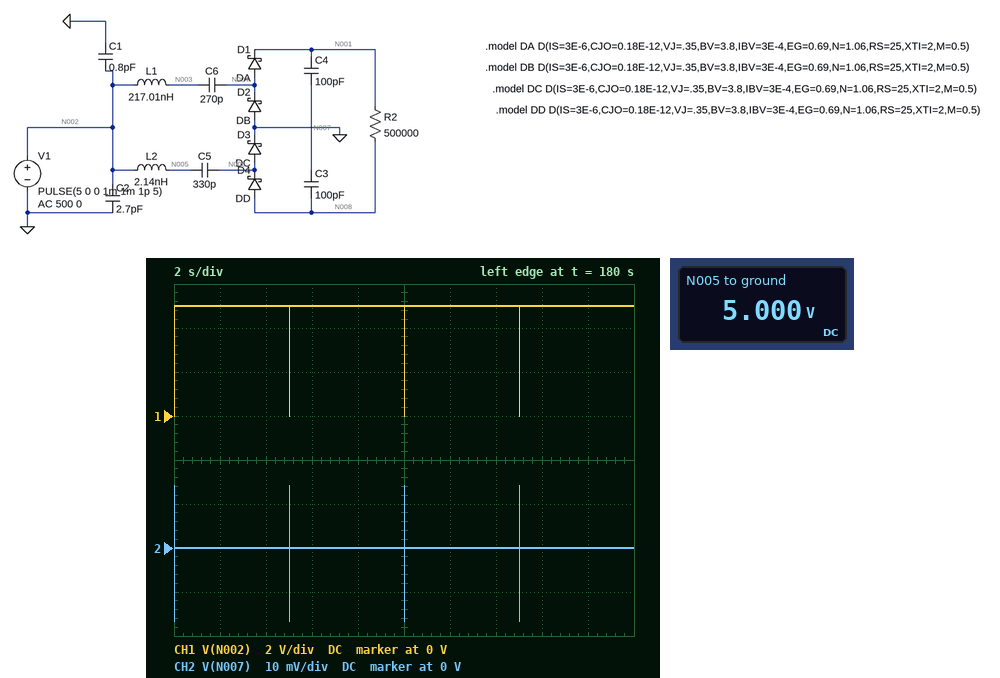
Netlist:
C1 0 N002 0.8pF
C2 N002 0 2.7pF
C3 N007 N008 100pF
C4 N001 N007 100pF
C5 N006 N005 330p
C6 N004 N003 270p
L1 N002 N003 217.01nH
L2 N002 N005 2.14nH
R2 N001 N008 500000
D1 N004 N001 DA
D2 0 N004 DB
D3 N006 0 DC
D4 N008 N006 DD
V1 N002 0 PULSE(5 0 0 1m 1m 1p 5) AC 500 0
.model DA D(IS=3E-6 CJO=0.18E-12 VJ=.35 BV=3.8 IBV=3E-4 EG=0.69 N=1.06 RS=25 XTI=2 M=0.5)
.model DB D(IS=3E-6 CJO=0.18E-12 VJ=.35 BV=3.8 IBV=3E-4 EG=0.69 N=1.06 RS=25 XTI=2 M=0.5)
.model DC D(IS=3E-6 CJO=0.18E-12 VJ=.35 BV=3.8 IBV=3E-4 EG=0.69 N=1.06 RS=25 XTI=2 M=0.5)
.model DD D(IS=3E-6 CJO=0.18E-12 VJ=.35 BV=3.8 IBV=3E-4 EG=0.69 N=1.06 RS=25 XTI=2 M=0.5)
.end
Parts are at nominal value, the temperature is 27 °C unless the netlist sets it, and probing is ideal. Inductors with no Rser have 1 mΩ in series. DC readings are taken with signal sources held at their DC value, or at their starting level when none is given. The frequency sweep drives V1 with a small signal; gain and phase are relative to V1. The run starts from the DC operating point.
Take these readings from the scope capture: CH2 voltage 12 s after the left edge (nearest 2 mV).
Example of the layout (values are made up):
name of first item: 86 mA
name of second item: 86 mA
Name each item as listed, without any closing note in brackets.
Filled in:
CH2 voltage 12 s after the left edge: 0 V
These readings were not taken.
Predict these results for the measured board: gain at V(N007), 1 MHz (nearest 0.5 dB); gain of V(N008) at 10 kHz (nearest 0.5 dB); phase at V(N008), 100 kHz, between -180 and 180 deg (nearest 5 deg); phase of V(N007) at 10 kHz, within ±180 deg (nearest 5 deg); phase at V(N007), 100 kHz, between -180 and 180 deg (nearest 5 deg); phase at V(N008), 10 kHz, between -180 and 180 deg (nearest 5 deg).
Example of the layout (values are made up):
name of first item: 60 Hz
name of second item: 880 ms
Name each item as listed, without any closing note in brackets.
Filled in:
gain at V(N007), 1 MHz: 0 dB
gain of V(N008) at 10 kHz: -14.5 dB
phase at V(N008), 100 kHz, between -180 and 180 deg: 30 deg
phase of V(N007) at 10 kHz, within ±180 deg: 80 deg
phase at V(N007), 100 kHz, between -180 and 180 deg: 30 deg
phase at V(N008), 10 kHz, between -180 and 180 deg: 80 deg
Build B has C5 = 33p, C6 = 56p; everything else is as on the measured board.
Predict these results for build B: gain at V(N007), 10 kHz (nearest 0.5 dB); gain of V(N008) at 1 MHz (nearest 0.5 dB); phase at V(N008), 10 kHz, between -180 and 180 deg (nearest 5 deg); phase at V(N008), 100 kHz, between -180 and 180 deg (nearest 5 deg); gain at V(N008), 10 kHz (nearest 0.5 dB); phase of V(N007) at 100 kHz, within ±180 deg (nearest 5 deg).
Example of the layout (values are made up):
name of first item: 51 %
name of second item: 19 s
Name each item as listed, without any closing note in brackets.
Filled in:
gain at V(N007), 10 kHz: -32.0 dB
gain of V(N008) at 1 MHz: -0.5 dB
phase at V(N008), 10 kHz, between -180 and 180 deg: 90 deg
phase at V(N008), 100 kHz, between -180 and 180 deg: 85 deg
gain at V(N008), 10 kHz: -34.0 dB
phase of V(N007) at 100 kHz, within ±180 deg: 75 deg
